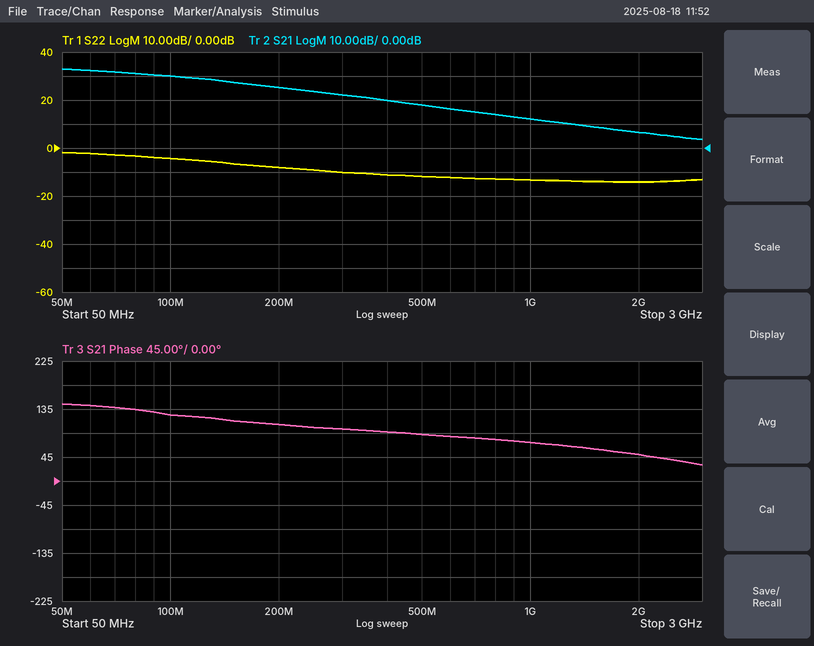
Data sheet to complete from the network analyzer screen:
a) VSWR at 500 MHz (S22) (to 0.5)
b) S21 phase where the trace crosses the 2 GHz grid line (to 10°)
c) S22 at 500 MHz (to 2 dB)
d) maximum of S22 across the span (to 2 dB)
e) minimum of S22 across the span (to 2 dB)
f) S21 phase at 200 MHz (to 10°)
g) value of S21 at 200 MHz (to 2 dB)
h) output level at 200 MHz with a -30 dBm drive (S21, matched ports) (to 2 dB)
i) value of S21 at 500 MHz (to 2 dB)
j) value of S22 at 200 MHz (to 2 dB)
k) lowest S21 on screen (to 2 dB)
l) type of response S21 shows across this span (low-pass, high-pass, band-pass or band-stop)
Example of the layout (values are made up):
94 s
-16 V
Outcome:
1.5
50°
-12 dB
-2 dB
-14 dB
110°
26 dB
-4 dBm
18 dB
-8 dB
4 dB
low-pass
